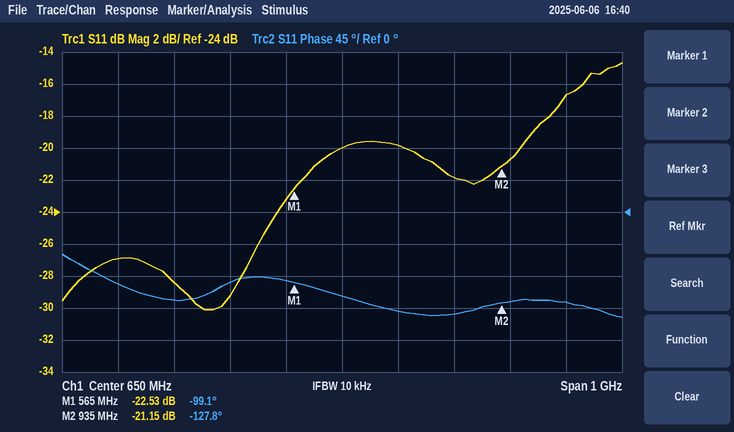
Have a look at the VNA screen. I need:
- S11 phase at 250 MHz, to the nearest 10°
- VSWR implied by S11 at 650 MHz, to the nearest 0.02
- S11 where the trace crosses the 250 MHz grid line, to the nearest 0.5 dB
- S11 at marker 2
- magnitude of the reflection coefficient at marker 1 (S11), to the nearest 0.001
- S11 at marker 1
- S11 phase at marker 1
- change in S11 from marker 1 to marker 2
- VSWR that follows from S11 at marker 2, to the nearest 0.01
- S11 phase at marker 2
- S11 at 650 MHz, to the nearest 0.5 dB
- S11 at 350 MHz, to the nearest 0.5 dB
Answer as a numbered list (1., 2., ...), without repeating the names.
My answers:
1. -100°
2. 1.22
3. -27.0 dB
4. -21.15 dB
5. 0.075
6. -22.53 dB
7. -99.1°
8. 1.38 dB
9. 1.19
10. -127.8°
11. -20.0 dB
12. -28.5 dB
